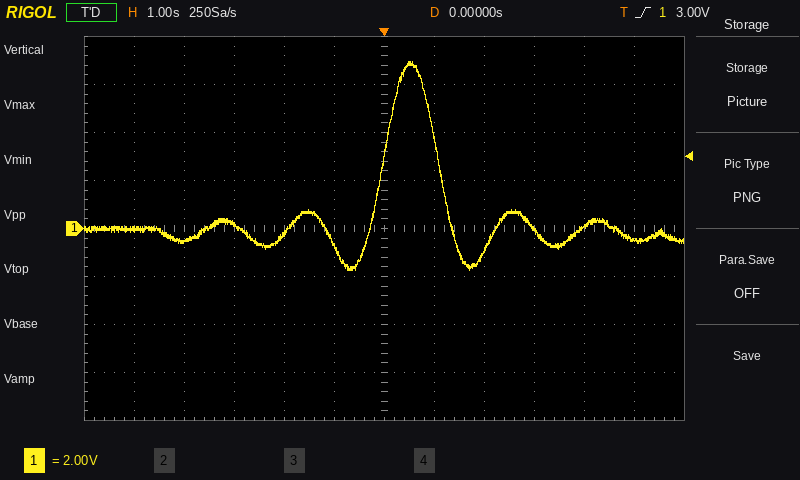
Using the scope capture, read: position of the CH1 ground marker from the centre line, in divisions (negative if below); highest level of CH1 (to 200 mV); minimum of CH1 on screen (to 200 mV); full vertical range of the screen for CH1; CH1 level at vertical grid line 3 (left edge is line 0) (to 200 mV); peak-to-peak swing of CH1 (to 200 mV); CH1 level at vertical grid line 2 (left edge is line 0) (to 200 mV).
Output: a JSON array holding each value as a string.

["0.0 div", "7.0 V", "-1.8 V", "16 V", "200 mV", "8.8 V", "-600 mV"]
